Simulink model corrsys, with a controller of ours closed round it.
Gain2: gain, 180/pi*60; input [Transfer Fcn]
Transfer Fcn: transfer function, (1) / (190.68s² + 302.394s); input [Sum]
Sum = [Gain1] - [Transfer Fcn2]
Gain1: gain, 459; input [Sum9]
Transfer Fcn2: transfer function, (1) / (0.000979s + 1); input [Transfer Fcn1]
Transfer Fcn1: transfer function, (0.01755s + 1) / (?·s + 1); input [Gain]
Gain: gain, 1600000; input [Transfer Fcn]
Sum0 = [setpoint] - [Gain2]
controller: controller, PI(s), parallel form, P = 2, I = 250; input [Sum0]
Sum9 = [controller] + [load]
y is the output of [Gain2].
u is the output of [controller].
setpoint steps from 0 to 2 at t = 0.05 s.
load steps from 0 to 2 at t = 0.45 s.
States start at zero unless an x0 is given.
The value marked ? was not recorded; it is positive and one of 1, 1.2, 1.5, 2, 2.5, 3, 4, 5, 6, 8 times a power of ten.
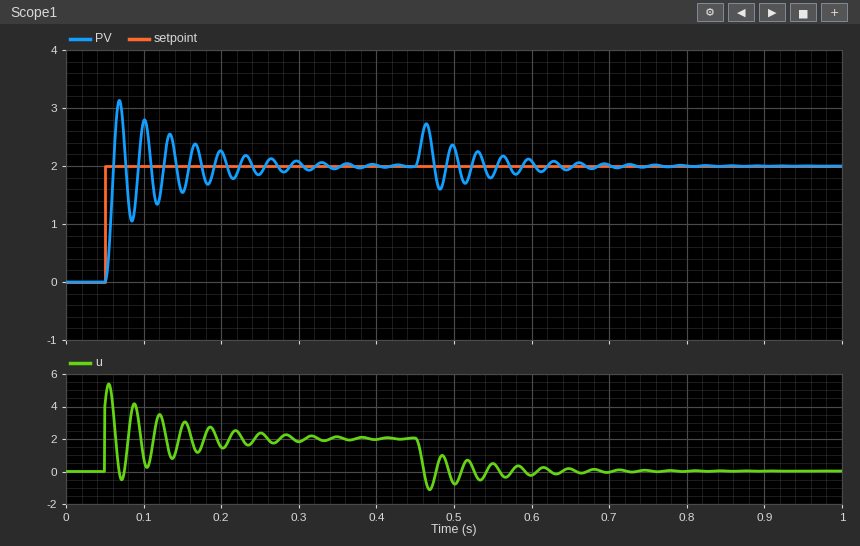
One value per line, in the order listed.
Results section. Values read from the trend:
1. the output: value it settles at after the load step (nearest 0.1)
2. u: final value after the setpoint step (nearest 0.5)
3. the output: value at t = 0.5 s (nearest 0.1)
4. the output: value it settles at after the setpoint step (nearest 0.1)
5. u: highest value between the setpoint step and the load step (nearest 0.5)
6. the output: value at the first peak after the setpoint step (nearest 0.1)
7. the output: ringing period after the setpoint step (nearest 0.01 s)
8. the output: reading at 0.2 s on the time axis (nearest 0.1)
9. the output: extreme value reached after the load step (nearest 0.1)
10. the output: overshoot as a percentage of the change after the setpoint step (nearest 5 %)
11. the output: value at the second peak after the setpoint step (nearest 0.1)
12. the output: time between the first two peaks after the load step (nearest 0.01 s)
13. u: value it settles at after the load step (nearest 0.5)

2.0
2.0
2.3
2.0
5.5
3.1
0.03 s
2.3
2.7
55 %
2.8
0.03 s
0.0
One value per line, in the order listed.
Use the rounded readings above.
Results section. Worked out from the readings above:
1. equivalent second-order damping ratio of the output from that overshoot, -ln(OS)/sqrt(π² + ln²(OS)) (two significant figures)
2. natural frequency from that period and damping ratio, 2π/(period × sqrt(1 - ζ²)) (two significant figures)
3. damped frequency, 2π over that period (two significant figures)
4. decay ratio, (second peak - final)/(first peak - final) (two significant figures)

0.19
210 rad/s
210 rad/s
0.73
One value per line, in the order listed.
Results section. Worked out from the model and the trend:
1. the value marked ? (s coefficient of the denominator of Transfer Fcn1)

0.003
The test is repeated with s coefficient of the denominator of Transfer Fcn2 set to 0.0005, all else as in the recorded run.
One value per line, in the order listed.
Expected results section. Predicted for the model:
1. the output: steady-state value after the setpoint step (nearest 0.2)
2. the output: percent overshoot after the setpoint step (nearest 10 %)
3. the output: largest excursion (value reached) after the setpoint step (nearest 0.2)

2.0
50 %
3.0
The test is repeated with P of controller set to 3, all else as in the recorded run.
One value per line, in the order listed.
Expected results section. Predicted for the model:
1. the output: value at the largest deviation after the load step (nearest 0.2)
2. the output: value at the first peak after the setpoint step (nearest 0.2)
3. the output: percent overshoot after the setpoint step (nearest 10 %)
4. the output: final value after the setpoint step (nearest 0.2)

2.6
3.0
50 %
2.0
